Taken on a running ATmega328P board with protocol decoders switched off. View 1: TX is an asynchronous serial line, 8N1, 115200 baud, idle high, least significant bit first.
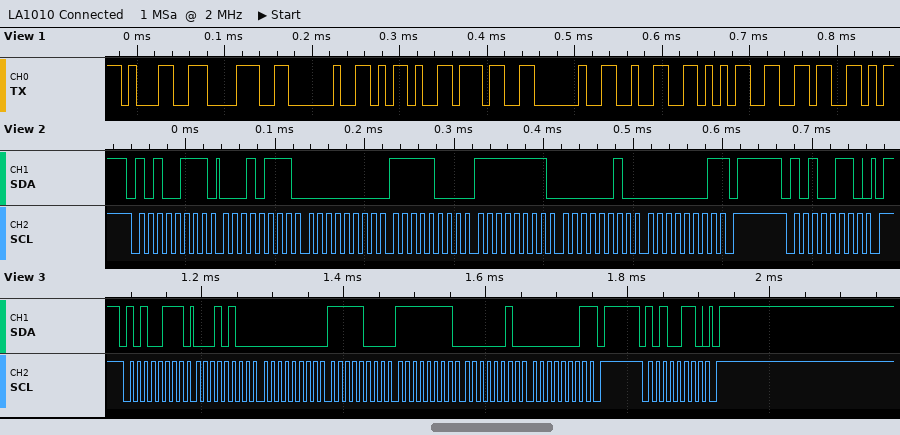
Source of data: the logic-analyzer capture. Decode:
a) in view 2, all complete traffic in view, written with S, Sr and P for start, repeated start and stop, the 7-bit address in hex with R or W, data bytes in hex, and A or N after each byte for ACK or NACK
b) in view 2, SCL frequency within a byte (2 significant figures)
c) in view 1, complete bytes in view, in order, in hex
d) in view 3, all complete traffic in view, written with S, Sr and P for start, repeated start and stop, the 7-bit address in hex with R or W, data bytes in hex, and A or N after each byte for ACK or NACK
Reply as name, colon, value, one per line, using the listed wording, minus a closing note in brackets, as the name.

in view 2, all complete traffic in view, written with S, Sr and P for start, repeated start and stop, the 7-bit address in hex with R or W, data bytes in hex, and A or N after each byte for ACK or NACK: S 53R A 17 A 00 A F8 A FF A 02 A 01 N P S 53W A P
in view 2, SCL frequency within a byte: 100 kHz
in view 1, complete bytes in view, in order, in hex: 31 38 20 2D 37 20 32 35 36
in view 3, all complete traffic in view, written with S, Sr and P for start, repeated start and stop, the 7-bit address in hex with R or W, data bytes in hex, and A or N after each byte for ACK or NACK: S 53R A 14 A 00 A F8 A FF A 02 A 01 N P S 53W A P
